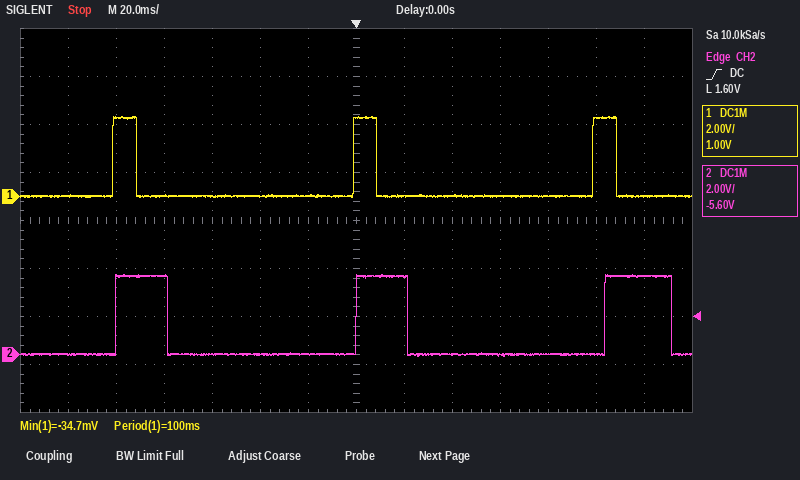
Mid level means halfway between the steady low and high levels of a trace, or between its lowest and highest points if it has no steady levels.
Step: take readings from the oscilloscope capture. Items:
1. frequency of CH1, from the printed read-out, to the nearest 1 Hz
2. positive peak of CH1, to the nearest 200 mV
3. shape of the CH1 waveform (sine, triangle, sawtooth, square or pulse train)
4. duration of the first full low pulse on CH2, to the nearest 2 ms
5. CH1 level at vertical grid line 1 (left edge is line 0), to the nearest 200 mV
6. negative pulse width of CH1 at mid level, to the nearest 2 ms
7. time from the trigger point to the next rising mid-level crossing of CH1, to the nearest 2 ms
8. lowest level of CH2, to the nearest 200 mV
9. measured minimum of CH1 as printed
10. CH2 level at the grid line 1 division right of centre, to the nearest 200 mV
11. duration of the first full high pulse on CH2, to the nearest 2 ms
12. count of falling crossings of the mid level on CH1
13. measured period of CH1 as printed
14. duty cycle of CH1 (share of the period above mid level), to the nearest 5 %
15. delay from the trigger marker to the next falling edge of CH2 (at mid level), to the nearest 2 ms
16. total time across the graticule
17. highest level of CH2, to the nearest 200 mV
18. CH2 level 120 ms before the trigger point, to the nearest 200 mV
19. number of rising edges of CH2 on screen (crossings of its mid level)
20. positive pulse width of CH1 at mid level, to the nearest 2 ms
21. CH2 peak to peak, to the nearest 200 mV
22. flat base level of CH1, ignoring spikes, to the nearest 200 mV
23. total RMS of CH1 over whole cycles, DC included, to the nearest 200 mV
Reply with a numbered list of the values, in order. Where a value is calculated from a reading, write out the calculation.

1. 1 / 100 ms ≈ 10 Hz
2. 3.4 V
3. pulse train
4. 78 ms
5. 0.0 V
6. 90 ms
7. 98 ms
8. 0.0 V
9. -34.7 mV
10. 3.2 V
11. 22 ms
12. 3
13. 100 ms
14. 10 %
15. 22 ms
16. 280 ms
17. 3.4 V
18. 0.0 V
19. 3
20. 10 ms
21. 3.4 V − (0.0 V) = 3.4 V
22. 0.0 V
23. √(0.1 × (3.4 V)² + 0.9 × (0.0 V)²) ≈ 1.08 V, so 1.0 V to the nearest 200 mV
